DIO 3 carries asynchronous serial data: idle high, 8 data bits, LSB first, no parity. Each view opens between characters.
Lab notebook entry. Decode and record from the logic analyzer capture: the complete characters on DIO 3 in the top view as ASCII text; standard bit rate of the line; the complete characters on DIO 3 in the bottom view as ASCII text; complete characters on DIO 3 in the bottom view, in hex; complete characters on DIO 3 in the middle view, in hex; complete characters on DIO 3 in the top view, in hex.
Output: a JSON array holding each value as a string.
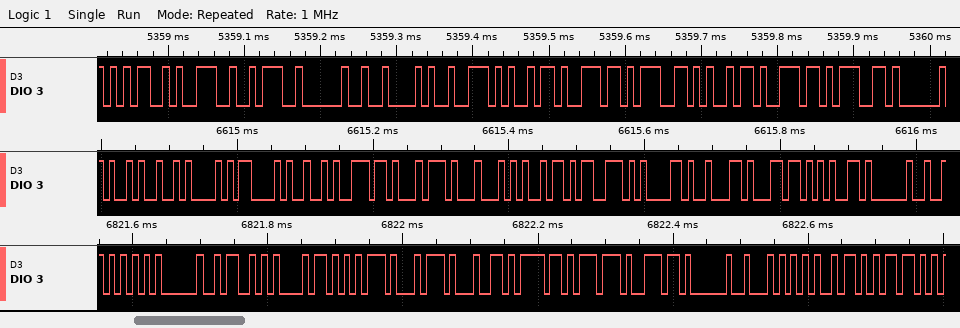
["\"59: Bringing\"", "115200 baud", "\"U Shutdown Tim\"", "55, 20, 53, 68, 75, 74, 64, 6F, 77, 6E, 20, 54, 69, 6D", "29, 0A, 0D, 49, 6E, 74, 44, 69, 73, 61, 62, 6C, 65, 20", "35, 39, 3A, 20, 42, 72, 69, 6E, 67, 69, 6E, 67"]
